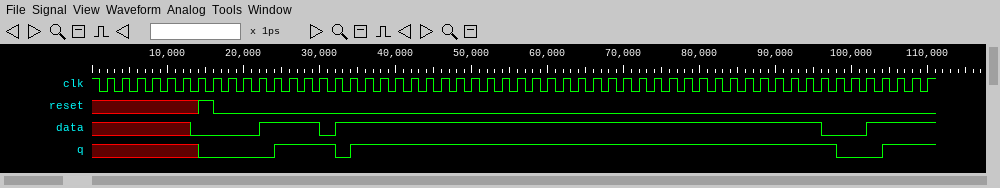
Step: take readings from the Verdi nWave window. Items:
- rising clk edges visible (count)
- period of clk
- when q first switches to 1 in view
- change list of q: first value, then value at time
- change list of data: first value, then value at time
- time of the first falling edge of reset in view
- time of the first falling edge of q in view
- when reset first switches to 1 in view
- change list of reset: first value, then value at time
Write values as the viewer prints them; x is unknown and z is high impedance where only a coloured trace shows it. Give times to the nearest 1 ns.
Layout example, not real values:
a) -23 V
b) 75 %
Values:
a) 55
b) 2 ns
c) 24 ns
d) x, 0 at 14 ns, 1 at 24 ns, 0 at 32 ns, 1 at 34 ns, 0 at 98 ns, 1 at 104 ns
e) x, 0 at 13 ns, 1 at 22 ns, 0 at 30 ns, 1 at 32 ns, 0 at 96 ns, 1 at 102 ns
f) 16 ns
g) 32 ns
h) 14 ns
i) x, 1 at 14 ns, 0 at 16 ns
